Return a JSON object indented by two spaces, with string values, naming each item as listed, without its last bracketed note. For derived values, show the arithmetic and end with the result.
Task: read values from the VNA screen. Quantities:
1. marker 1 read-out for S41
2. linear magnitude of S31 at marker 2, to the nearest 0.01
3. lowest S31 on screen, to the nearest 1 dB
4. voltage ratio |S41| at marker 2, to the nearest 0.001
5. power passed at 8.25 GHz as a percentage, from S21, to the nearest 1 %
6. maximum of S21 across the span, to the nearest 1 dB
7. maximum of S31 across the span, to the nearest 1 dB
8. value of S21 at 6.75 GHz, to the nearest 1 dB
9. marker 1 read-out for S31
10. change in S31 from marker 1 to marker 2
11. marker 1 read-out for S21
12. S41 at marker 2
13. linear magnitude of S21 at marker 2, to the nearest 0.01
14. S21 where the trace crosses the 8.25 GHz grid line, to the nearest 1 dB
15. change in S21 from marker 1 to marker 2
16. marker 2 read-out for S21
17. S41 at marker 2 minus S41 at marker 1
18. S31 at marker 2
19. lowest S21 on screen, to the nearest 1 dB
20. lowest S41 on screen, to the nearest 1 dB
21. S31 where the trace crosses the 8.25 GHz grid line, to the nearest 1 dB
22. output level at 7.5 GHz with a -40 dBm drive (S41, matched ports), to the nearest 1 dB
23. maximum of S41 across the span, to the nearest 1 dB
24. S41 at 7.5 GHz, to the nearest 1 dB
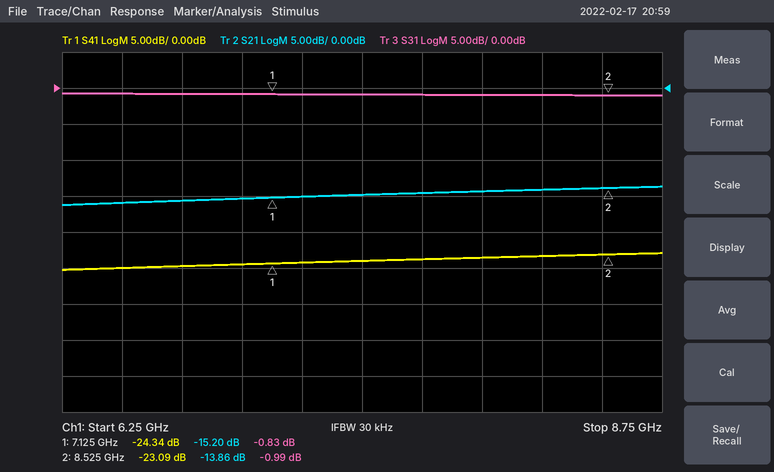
{
  "marker 1 read-out for S41": "-24.34 dB",
  "linear magnitude of S31 at marker 2, to the nearest 0.01": "10^(-0.99/20) ≈ 0.89",
  "lowest S31 on screen, to the nearest 1 dB": "-1 dB",
  "voltage ratio |S41| at marker 2, to the nearest 0.001": "10^(-23.09/20) ≈ 0.070",
  "power passed at 8.25 GHz as a percentage, from S21, to the nearest 1 %": "10^(-14/10) ≈ 4 %",
  "maximum of S21 across the span, to the nearest 1 dB": "-14 dB",
  "maximum of S31 across the span, to the nearest 1 dB": "-1 dB",
  "value of S21 at 6.75 GHz, to the nearest 1 dB": "-16 dB",
  "marker 1 read-out for S31": "-0.83 dB",
  "change in S31 from marker 1 to marker 2": "-0.99 − (-0.83) = -0.16 dB",
  "marker 1 read-out for S21": "-15.20 dB",
  "S41 at marker 2": "-23.09 dB",
  "linear magnitude of S21 at marker 2, to the nearest 0.01": "10^(-13.86/20) ≈ 0.20",
  "S21 where the trace crosses the 8.25 GHz grid line, to the nearest 1 dB": "-14 dB",
  "change in S21 from marker 1 to marker 2": "-13.86 − (-15.2) = 1.34 dB",
  "marker 2 read-out for S21": "-13.86 dB",
  "S41 at marker 2 minus S41 at marker 1": "-23.09 − (-24.34) = 1.25 dB",
  "S31 at marker 2": "-0.99 dB",
  "lowest S21 on screen, to the nearest 1 dB": "-16 dB",
  "lowest S41 on screen, to the nearest 1 dB": "-25 dB",
  "S31 where the trace crosses the 8.25 GHz grid line, to the nearest 1 dB": "-1 dB",
  "output level at 7.5 GHz with a -40 dBm drive (S41, matched ports), to the nearest 1 dB": "-40 dBm + (-24 dB) = -64 dBm",
  "maximum of S41 across the span, to the nearest 1 dB": "-23 dB",
  "S41 at 7.5 GHz, to the nearest 1 dB": "-24 dB"
}
